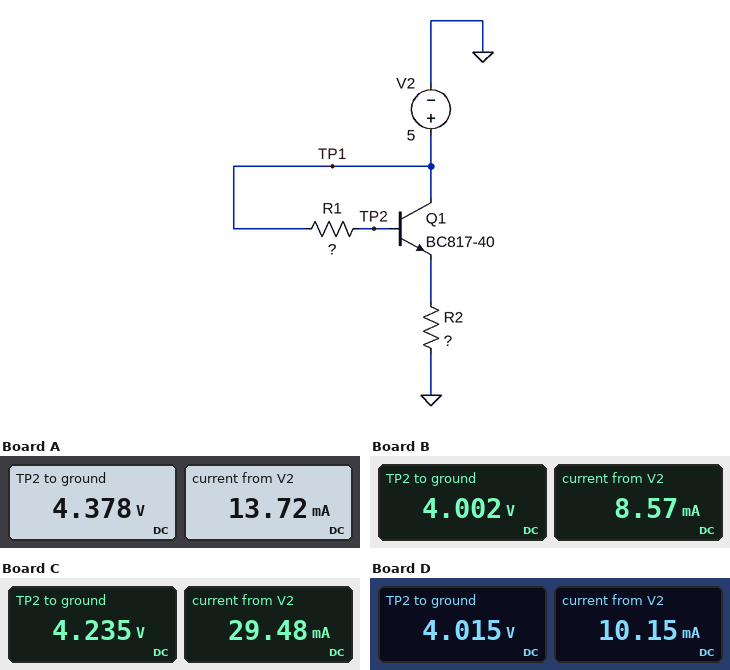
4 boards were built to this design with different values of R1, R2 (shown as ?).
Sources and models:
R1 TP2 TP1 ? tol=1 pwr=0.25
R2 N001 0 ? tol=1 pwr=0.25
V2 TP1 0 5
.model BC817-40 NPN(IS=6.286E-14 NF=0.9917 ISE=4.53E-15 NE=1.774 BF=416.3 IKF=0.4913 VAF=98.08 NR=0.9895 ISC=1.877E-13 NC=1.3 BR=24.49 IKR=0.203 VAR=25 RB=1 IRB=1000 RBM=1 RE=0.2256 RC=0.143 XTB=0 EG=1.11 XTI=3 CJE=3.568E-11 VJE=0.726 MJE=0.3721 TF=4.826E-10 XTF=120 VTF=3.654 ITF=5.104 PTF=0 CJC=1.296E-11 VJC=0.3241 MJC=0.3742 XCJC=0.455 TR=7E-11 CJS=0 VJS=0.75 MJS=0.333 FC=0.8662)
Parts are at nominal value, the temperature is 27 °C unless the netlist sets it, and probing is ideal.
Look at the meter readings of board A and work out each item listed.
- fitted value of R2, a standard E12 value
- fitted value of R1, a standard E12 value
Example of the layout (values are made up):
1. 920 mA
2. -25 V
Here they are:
1. 270 Ω
2. 18 kΩ
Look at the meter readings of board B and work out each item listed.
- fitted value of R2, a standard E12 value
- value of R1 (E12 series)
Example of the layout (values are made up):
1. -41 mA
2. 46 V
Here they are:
1. 390 Ω
2. 47 kΩ
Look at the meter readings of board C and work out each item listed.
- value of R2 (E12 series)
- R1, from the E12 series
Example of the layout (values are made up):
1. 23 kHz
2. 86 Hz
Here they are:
1. 120 Ω
2. 10 kΩ
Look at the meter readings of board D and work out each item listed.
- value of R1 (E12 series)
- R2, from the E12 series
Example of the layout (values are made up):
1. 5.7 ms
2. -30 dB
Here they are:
1. 39 kΩ
2. 330 Ω
